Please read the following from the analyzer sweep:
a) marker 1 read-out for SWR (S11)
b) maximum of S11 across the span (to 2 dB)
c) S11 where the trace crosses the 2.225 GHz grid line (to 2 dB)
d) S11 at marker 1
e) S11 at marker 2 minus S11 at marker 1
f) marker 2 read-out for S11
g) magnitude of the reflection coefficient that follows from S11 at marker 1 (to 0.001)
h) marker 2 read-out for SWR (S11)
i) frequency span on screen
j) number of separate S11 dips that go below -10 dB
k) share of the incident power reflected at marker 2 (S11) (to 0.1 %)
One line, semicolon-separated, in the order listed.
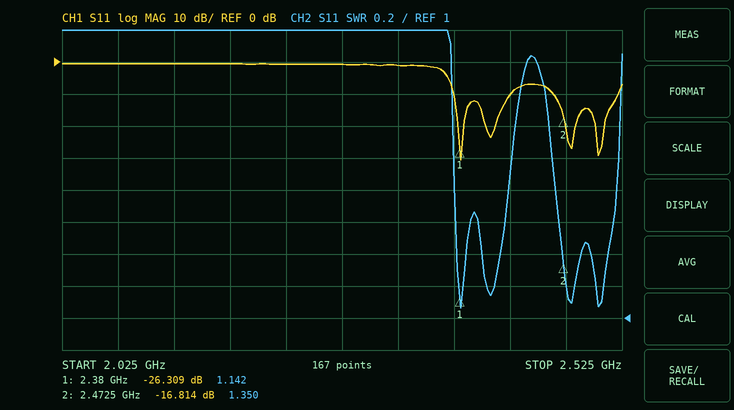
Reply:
1.142; 0 dB; 0 dB; -26.309 dB; 9.495 dB; -16.814 dB; 0.048; 1.350; 500 MHz; 4; 2.1 %
